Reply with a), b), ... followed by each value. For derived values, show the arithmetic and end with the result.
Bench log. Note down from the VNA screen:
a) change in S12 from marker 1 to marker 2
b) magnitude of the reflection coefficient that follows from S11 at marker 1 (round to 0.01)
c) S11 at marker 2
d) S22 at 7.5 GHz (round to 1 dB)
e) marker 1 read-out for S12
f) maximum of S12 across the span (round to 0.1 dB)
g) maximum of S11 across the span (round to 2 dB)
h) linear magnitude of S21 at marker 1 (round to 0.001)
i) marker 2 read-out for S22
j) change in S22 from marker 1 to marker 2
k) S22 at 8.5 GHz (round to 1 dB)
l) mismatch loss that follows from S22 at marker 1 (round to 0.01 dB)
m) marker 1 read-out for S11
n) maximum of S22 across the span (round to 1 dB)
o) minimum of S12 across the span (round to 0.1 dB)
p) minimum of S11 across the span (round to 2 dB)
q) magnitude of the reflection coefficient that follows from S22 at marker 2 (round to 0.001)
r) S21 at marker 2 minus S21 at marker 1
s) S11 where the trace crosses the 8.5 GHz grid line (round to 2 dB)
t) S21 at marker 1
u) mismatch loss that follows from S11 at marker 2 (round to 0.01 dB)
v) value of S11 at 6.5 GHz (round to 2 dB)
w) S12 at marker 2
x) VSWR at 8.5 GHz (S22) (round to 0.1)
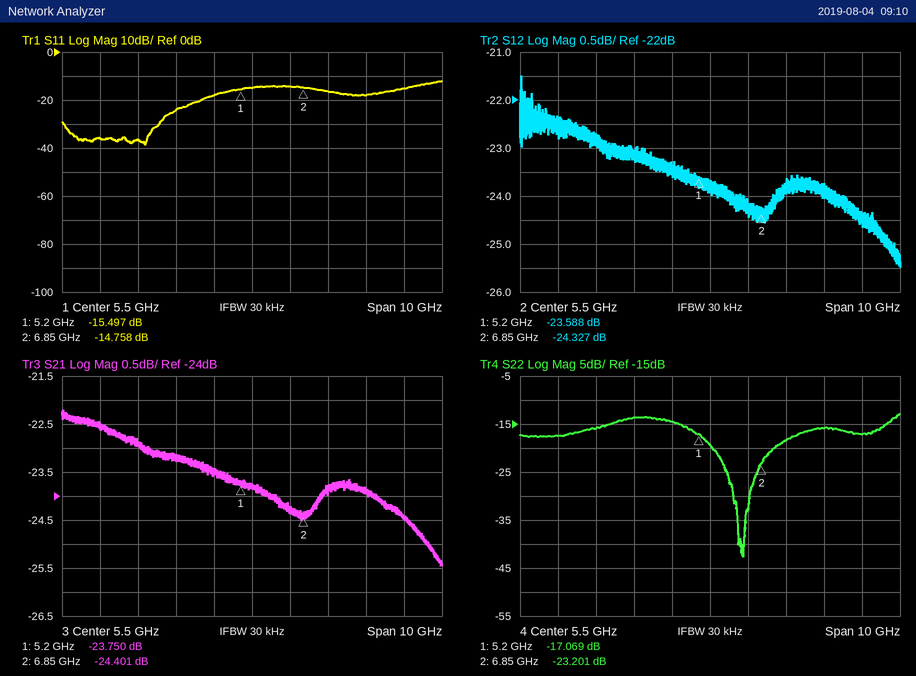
a) -24.327 − (-23.588) = -0.739 dB
b) 10^(-15.497/20) ≈ 0.17
c) -14.758 dB
d) -18 dB
e) -23.588 dB
f) -21.5 dB
g) -12 dB
h) 10^(-23.75/20) ≈ 0.065
i) -23.201 dB
j) -23.201 − (-17.069) = -6.132 dB
k) -16 dB
l) −10 log10(1 − 10^(-17.069/10)) ≈ 0.09 dB
m) -15.497 dB
n) -13 dB
o) -25.5 dB
p) -38 dB
q) 10^(-23.201/20) ≈ 0.069
r) -24.401 − (-23.75) = -0.651 dB
s) -18 dB
t) -23.750 dB
u) −10 log10(1 − 10^(-14.758/10)) ≈ 0.15 dB
v) -14 dB
w) -24.327 dB
x) |Γ| = 10^(-16/20) = 0.1585; VSWR = (1 + 0.1585)/(1 − 0.1585) ≈ 1.4
